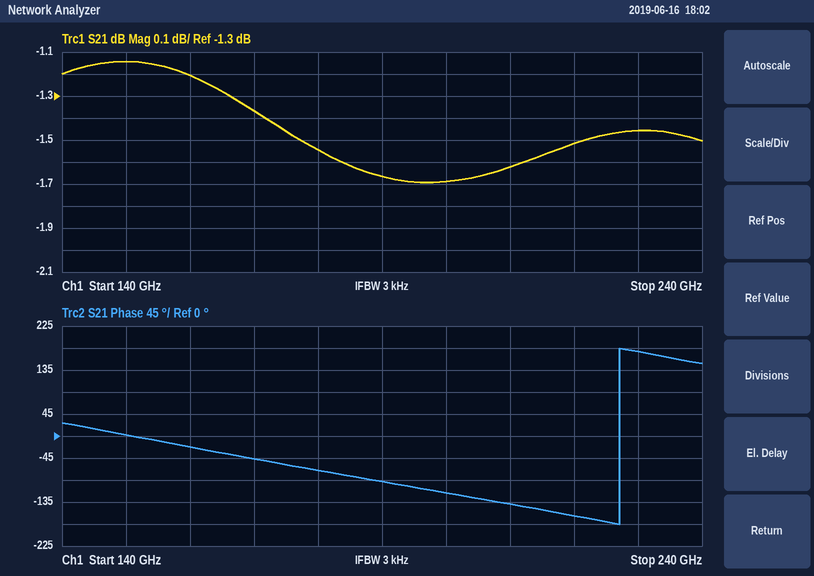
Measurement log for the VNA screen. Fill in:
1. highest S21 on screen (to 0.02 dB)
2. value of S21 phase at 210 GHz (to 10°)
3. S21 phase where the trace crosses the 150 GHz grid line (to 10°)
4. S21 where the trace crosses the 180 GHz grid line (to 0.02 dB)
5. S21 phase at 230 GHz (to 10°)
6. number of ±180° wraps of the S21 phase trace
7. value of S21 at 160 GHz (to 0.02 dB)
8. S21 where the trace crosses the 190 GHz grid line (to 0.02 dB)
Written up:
-1.14 dB
-140°
0°
-1.54 dB
170°
1
-1.20 dB
-1.66 dB
